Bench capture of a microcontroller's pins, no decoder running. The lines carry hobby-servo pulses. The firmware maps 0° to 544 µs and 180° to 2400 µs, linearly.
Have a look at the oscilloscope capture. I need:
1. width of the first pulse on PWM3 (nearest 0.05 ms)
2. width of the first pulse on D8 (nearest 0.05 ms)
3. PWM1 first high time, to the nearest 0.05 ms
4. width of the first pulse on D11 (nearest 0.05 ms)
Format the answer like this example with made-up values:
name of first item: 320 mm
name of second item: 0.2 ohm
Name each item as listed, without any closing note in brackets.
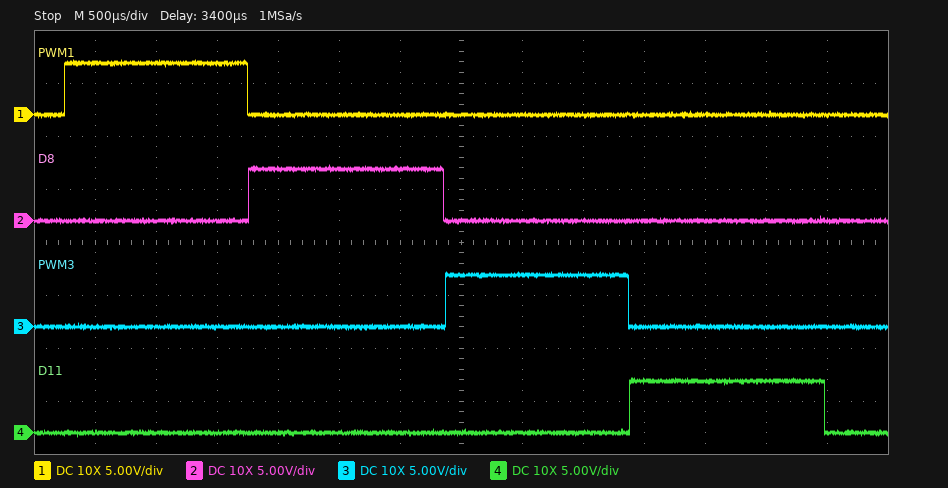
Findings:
width of the first pulse on PWM3: 1.50 ms
width of the first pulse on D8: 1.60 ms
PWM1 first high time, to the nearest 0.05 ms: 1.50 ms
width of the first pulse on D11: 1.60 ms
